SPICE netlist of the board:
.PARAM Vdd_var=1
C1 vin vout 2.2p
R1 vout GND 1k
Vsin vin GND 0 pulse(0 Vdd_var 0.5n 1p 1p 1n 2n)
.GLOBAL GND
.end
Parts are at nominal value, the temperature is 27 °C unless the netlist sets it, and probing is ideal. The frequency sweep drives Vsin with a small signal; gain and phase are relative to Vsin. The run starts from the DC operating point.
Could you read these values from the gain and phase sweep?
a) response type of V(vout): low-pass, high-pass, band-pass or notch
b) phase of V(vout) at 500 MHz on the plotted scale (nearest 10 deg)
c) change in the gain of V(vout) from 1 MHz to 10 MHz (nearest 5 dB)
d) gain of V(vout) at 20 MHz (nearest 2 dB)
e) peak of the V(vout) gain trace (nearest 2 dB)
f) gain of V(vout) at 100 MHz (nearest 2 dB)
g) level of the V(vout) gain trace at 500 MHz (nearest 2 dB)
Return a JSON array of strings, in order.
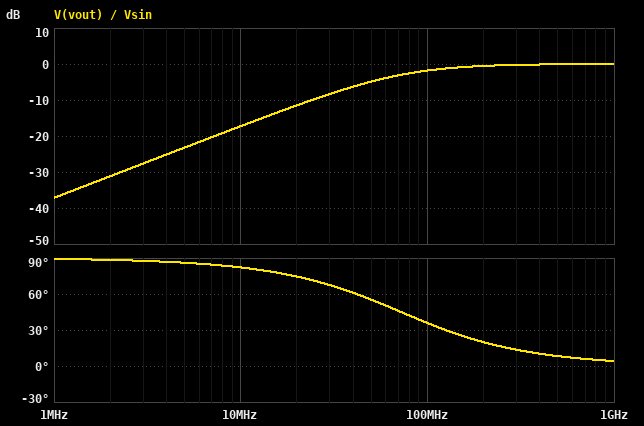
["high-pass", "10 deg", "20 dB", "-12 dB", "0 dB", "-2 dB", "0 dB"]
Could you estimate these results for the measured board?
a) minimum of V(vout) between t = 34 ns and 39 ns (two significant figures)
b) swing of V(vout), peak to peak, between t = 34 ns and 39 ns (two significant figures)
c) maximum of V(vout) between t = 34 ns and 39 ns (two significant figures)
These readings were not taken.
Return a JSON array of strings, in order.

["-610 mV", "1.2 V", "610 mV"]
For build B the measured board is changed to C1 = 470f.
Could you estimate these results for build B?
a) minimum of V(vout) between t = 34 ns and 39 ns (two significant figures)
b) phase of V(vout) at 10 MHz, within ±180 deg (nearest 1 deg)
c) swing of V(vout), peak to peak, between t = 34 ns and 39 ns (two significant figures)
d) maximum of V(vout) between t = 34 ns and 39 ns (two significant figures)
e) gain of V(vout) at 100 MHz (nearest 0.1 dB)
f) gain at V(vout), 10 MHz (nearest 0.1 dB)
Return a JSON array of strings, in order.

["-890 mV", "88 deg", "1.8 V", "890 mV", "-11.0 dB", "-30.6 dB"]
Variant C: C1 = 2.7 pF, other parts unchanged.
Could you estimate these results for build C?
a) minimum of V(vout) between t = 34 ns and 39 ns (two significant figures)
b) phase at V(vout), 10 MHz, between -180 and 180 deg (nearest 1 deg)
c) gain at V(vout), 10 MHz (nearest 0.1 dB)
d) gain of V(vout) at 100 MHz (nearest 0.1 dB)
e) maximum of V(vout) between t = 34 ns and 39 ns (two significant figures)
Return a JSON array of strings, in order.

["-590 mV", "80 deg", "-15.5 dB", "-1.3 dB", "590 mV"]
